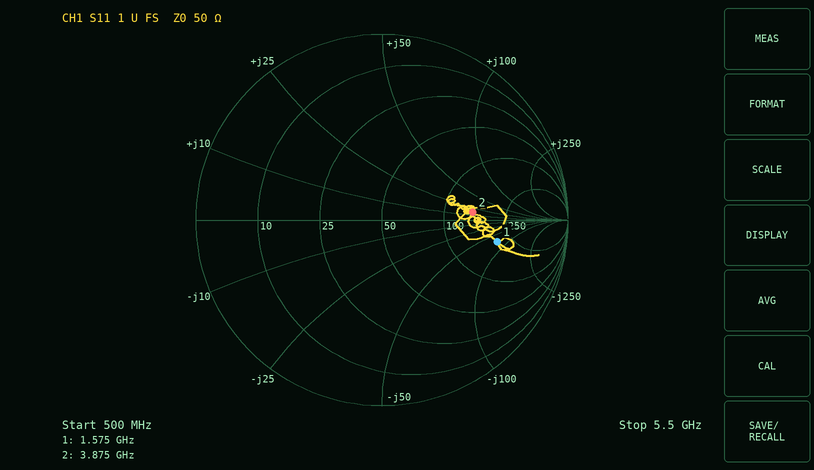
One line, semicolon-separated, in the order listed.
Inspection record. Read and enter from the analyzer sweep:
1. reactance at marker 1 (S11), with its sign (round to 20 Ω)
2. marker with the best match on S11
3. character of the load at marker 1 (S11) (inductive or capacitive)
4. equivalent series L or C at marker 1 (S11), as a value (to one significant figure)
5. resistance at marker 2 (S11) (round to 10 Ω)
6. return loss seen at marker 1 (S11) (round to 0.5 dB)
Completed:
-80 Ω; marker 2; capacitive; 1 pF; 140 Ω; 4.0 dB
